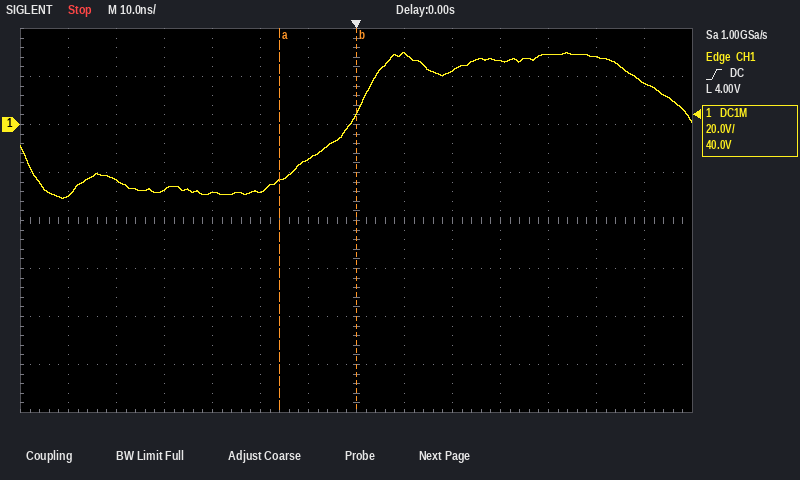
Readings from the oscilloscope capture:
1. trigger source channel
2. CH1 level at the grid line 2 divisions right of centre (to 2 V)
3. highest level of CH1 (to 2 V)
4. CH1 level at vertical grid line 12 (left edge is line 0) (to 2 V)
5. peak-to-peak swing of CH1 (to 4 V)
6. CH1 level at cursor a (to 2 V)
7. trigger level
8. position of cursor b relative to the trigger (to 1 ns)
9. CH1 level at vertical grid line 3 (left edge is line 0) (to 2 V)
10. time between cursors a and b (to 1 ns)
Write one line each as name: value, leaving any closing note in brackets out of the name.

trigger source channel: CH1
CH1 level at the grid line 2 divisions right of centre: 22 V
highest level of CH1: 30 V
CH1 level at vertical grid line 12 (left edge is line 0): 28 V
peak-to-peak swing of CH1: 60 V
CH1 level at cursor a: -24 V
trigger level: 4.00 V
position of cursor b relative to the trigger: 0 ns
CH1 level at vertical grid line 3 (left edge is line 0): -28 V
time between cursors a and b: 16 ns
